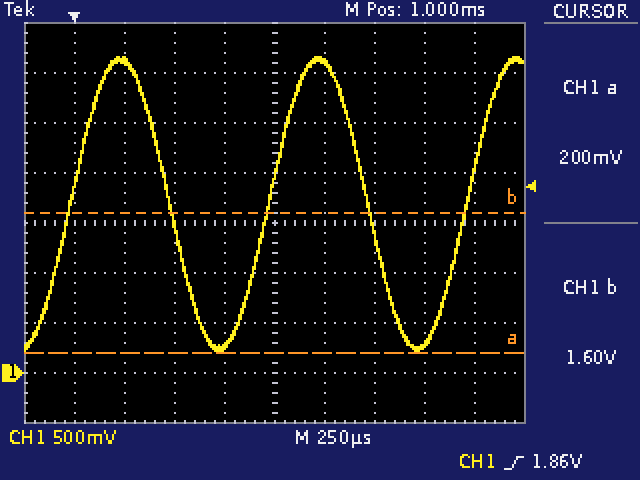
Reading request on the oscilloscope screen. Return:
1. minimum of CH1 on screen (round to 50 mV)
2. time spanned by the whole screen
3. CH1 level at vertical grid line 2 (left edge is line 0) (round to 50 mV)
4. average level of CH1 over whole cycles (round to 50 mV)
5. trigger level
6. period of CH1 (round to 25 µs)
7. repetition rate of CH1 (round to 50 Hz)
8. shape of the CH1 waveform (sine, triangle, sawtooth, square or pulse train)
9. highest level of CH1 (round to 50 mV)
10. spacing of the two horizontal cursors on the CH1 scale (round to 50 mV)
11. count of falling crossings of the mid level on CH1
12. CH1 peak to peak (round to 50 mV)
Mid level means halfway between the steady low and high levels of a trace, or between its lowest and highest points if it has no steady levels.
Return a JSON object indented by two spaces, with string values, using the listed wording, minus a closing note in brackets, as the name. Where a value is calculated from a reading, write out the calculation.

{
  "minimum of CH1 on screen": "200 mV",
  "time spanned by the whole screen": "2.5 ms",
  "CH1 level at vertical grid line 2 (left edge is line 0)": "3.10 V",
  "average level of CH1 over whole cycles": "(3.15 V + (200 mV)) / 2 ≈ 1.68 V, so 1.70 V to the nearest 50 mV",
  "trigger level": "1.86 V",
  "period of CH1": "1.000 ms",
  "repetition rate of CH1": "1 / 1.000 ms ≈ 1.00 kHz",
  "shape of the CH1 waveform": "sine",
  "highest level of CH1": "3.15 V",
  "spacing of the two horizontal cursors on the CH1 scale": "1.40 V",
  "count of falling crossings of the mid level on CH1": "2",
  "CH1 peak to peak": "3.15 V − (200 mV) = 2.95 V"
}
